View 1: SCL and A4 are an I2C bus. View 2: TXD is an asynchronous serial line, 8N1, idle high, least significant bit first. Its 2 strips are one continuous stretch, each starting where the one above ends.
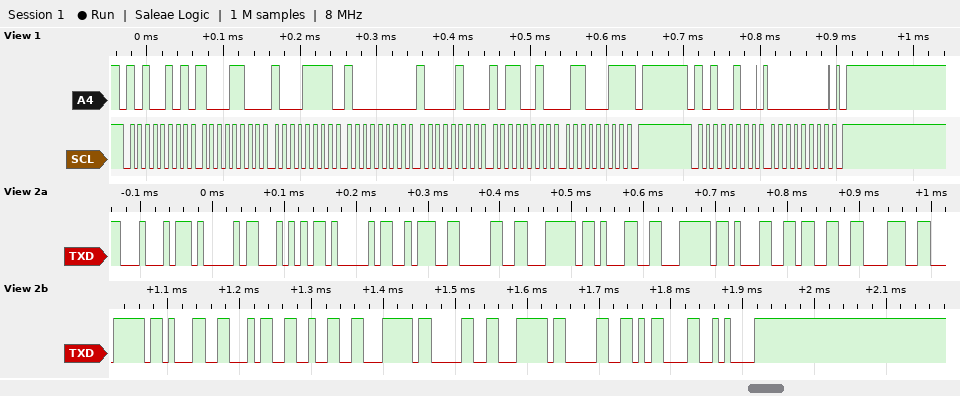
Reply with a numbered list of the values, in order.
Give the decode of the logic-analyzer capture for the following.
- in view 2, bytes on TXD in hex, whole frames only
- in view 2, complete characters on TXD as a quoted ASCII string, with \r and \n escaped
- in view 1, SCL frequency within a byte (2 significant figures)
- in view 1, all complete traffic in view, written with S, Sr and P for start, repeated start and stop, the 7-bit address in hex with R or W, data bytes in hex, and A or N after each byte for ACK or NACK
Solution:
1. 44 41 54 41 3A 30 7C 31 7C 31 33 38 7C 31 34 32 7C 30 7C 30 0D 0A
2. "DATA:0|1|138|142|0|0\r\n"
3. 100 kHz
4. S 52R A 8C A 8F A 80 A 84 A B2 A 63 N P S 52W A 00 A P
